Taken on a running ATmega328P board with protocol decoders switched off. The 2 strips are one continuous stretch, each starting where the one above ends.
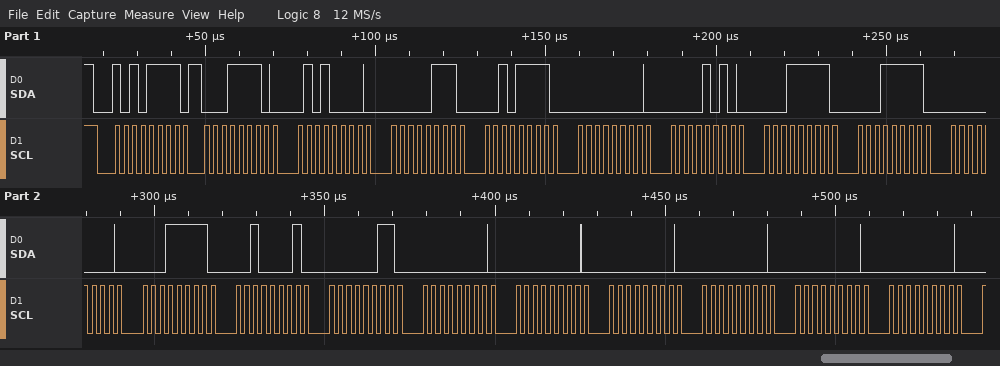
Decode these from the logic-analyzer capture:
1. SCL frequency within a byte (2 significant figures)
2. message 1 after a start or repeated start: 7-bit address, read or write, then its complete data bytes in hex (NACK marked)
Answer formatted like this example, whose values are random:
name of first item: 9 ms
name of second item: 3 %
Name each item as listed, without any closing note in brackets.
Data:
SCL frequency within a byte: 400 kHz
message 1 after a start or repeated start: 7-bit address, read or write, then its complete data bytes in hex: 0x57 read: 1E 50 07 2F 00 0A 1F 1F 00 1F 21 03 00 00 00 00 00 00
